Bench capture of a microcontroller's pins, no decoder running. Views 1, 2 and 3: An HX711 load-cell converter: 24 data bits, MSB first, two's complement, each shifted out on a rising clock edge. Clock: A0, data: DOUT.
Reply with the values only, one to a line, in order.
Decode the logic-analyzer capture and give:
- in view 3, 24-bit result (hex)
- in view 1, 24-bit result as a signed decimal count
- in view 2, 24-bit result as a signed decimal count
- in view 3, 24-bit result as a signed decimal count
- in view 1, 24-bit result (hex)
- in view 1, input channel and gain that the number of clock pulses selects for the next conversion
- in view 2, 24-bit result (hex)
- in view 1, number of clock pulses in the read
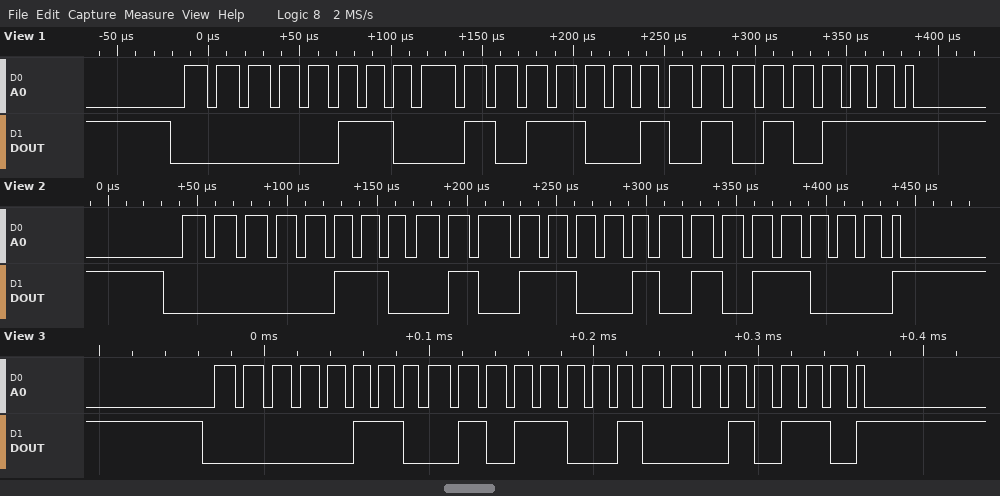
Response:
0x065916
416087
416088
416022
0x065957
channel A, gain 128
0x065958
25
